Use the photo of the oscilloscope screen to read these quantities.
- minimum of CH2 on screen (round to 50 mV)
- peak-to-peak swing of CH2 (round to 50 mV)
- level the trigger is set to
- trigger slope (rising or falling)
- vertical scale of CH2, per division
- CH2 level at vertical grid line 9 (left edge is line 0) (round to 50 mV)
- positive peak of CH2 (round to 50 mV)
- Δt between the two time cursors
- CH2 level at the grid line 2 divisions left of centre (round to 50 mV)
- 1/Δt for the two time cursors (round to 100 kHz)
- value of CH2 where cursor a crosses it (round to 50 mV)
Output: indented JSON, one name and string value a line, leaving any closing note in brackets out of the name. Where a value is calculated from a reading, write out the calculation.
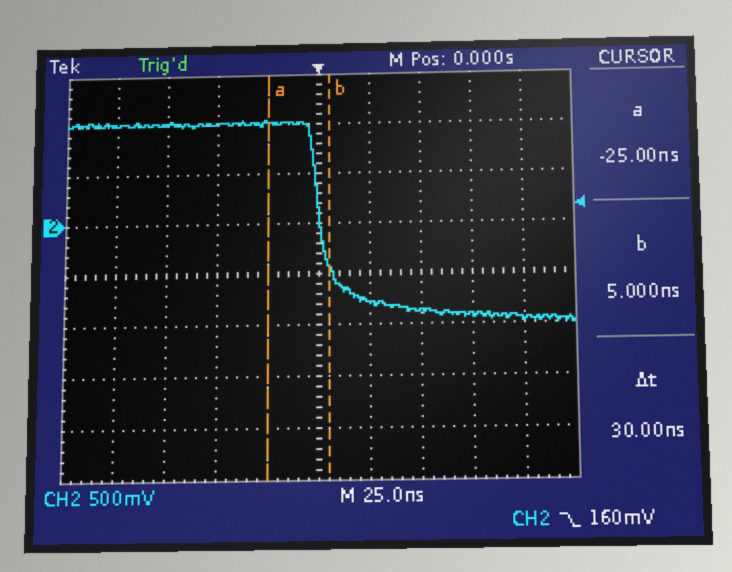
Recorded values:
{
  "minimum of CH2 on screen": "-1.00 V",
  "peak-to-peak swing of CH2": "1.05 V − (-1.00 V) = 2.05 V",
  "level the trigger is set to": "160 mV",
  "trigger slope": "falling",
  "vertical scale of CH2, per division": "500 mV",
  "CH2 level at vertical grid line 9 (left edge is line 0)": "-950 mV",
  "positive peak of CH2": "1.05 V",
  "Δt between the two time cursors": "30 ns",
  "CH2 level at the grid line 2 divisions left of centre": "1.00 V",
  "1/Δt for the two time cursors": "1 / 30 ns ≈ 33.3 MHz",
  "value of CH2 where cursor a crosses it": "1.00 V"
}
